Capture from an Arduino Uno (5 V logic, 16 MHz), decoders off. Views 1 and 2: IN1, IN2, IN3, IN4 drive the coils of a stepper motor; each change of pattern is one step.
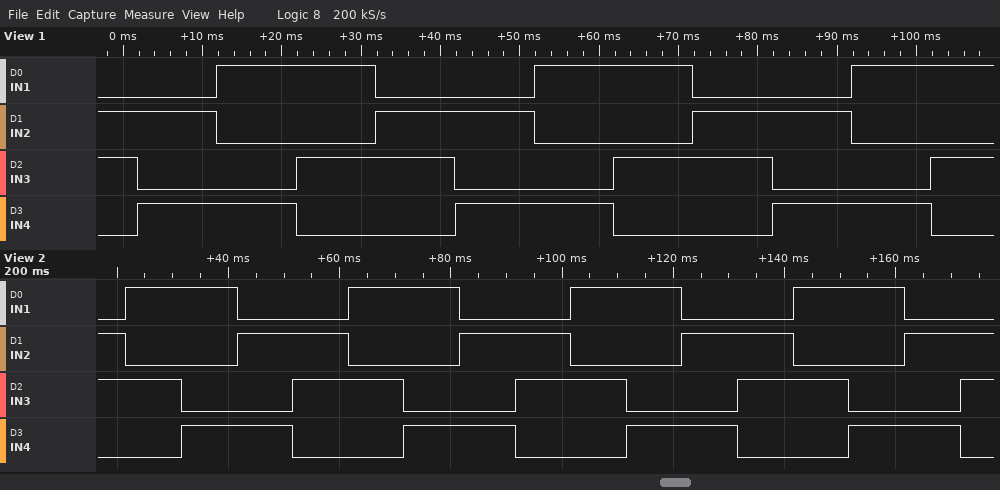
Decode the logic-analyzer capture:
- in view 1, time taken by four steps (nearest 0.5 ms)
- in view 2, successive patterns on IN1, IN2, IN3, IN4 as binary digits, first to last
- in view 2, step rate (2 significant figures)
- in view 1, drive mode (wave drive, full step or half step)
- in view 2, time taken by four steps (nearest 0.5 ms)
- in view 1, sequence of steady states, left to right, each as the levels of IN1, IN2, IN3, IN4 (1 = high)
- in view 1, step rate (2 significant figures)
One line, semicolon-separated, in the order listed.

40.0 ms; 0110 1010 1001 0101 0110 1010 1001 0101 0110 1010 1001 0101 0110 1010 1001 0101 0110; 100 steps/s; full step; 40.0 ms; 0110 0101 1001 1010 0110 0101 1001 1010 0110 0101 1001 1010; 100 steps/s
